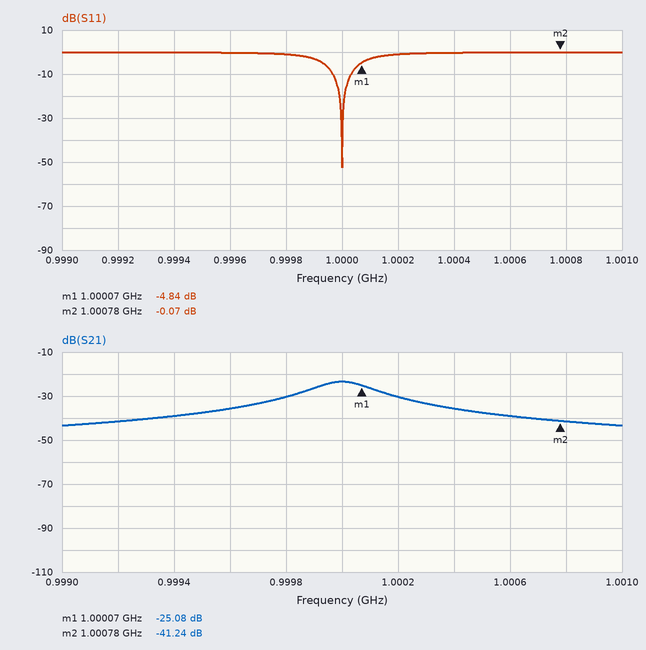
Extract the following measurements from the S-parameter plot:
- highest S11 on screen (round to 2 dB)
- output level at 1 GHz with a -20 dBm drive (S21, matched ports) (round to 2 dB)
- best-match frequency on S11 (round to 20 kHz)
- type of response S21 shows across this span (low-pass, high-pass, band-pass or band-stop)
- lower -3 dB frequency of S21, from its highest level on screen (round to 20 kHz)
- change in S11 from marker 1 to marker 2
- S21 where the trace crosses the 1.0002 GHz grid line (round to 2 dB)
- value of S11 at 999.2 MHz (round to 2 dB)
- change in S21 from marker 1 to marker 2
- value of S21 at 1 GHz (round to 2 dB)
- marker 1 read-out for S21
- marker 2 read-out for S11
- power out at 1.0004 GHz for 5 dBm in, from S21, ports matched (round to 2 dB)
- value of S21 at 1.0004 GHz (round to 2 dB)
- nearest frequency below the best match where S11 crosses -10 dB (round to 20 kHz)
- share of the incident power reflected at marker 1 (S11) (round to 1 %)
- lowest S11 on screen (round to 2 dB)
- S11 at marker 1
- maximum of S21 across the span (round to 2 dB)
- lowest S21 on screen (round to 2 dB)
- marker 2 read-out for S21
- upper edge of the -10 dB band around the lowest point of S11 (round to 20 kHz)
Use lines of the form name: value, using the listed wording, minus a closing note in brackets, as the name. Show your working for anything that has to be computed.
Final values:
highest S11 on screen: 0 dB
output level at 1 GHz with a -20 dBm drive (S21, matched ports): -20 dBm + (-24 dB) = -44 dBm
best-match frequency on S11: 1.00000 GHz
type of response S21 shows across this span: band-pass
lower -3 dB frequency of S21, from its highest level on screen: 999.90 MHz
change in S11 from marker 1 to marker 2: -0.07 − (-4.84) = 4.77 dB
S21 where the trace crosses the 1.0002 GHz grid line: -30 dB
value of S11 at 999.2 MHz: 0 dB
change in S21 from marker 1 to marker 2: -41.24 − (-25.08) = -16.16 dB
value of S21 at 1 GHz: -24 dB
marker 1 read-out for S21: -25.08 dB
marker 2 read-out for S11: -0.07 dB
power out at 1.0004 GHz for 5 dBm in, from S21, ports matched: 5 dBm + (-36 dB) = -30 dBm
value of S21 at 1.0004 GHz: -36 dB
nearest frequency below the best match where S11 crosses -10 dB: 999.96 MHz
share of the incident power reflected at marker 1 (S11): 10^(-4.84/10) ≈ 33 %
lowest S11 on screen: -52 dB
S11 at marker 1: -4.84 dB
maximum of S21 across the span: -24 dB
lowest S21 on screen: -44 dB
marker 2 read-out for S21: -41.24 dB
upper edge of the -10 dB band around the lowest point of S11: 1.00004 GHz
